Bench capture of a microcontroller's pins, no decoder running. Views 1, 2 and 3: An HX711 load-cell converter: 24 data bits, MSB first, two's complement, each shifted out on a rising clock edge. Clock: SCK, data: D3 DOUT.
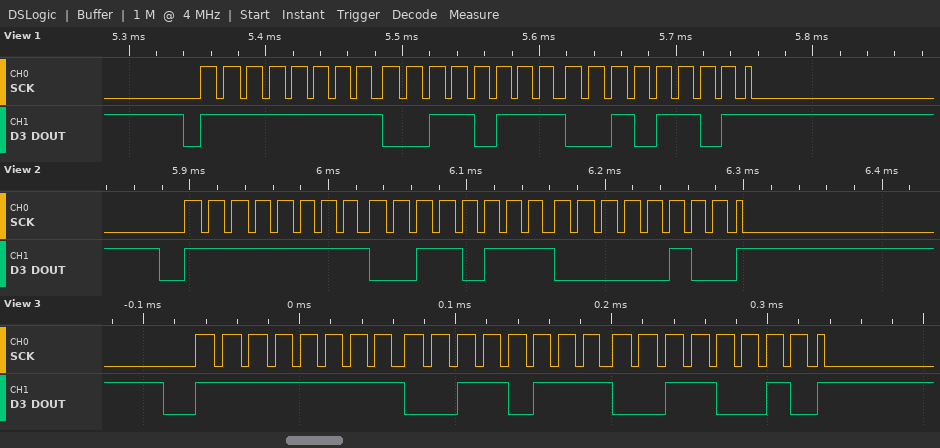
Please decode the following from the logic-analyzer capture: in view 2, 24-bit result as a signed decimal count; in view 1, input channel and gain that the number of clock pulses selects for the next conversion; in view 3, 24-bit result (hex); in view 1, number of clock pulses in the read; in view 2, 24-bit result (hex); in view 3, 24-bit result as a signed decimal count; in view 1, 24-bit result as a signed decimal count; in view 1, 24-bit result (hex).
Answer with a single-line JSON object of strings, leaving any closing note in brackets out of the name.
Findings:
{"in view 2, 24-bit result as a signed decimal count": "-51452", "in view 1, input channel and gain that the number of clock pulses selects for the next conversion": "channel A, gain 128", "in view 3, 24-bit result": "0xFF3732", "in view 1, number of clock pulses in the read": "25", "in view 2, 24-bit result": "0xFF3704", "in view 3, 24-bit result as a signed decimal count": "-51406", "in view 1, 24-bit result as a signed decimal count": "-51411", "in view 1, 24-bit result": "0xFF372D"}
